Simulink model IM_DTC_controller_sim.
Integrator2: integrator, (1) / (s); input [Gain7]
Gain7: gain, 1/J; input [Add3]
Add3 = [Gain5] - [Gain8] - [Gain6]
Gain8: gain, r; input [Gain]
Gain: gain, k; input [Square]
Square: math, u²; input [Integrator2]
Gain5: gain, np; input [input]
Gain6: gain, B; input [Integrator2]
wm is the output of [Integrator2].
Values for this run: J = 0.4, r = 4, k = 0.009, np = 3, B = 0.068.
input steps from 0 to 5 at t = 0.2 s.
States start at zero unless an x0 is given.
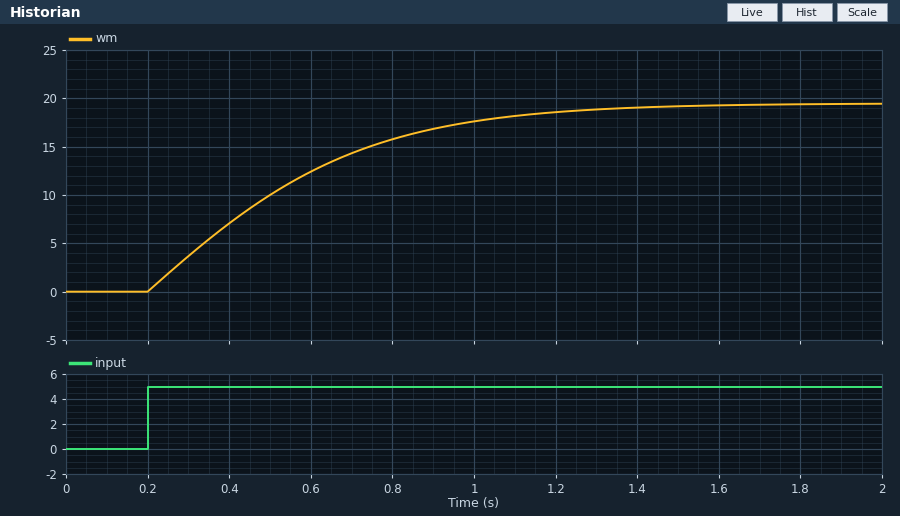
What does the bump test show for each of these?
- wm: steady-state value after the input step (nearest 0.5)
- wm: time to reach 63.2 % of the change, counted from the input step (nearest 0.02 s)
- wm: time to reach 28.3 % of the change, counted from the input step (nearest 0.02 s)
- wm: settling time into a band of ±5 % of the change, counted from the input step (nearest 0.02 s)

19.5
0.40 s
0.16 s
0.98 s
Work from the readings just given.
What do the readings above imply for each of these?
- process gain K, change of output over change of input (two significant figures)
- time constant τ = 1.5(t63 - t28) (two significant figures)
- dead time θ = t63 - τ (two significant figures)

3.9
0.36 s
0.040 s
